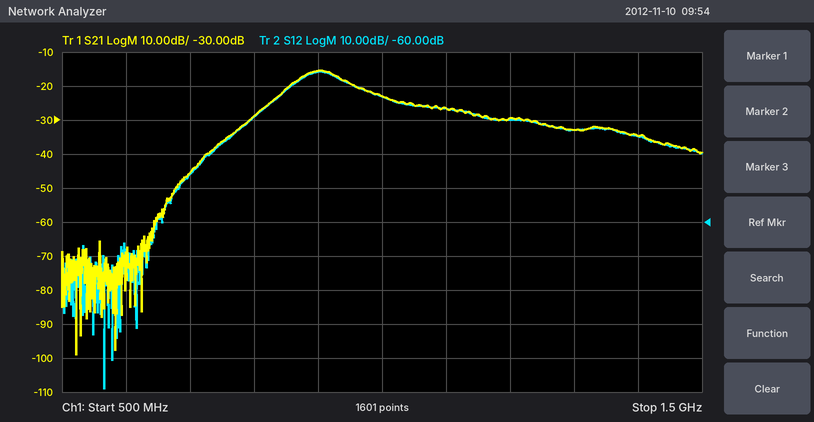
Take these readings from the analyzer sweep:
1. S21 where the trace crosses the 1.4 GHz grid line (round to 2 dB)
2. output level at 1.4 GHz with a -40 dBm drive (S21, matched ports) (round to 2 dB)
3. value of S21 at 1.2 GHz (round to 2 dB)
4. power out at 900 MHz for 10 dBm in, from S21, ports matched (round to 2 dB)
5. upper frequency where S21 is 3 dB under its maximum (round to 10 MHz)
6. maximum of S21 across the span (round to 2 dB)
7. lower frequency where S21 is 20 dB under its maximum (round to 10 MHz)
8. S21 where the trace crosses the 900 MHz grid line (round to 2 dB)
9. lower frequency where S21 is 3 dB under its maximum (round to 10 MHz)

-34 dB
-74 dBm
-30 dB
-6 dBm
940 MHz
-16 dB
760 MHz
-16 dB
870 MHz
